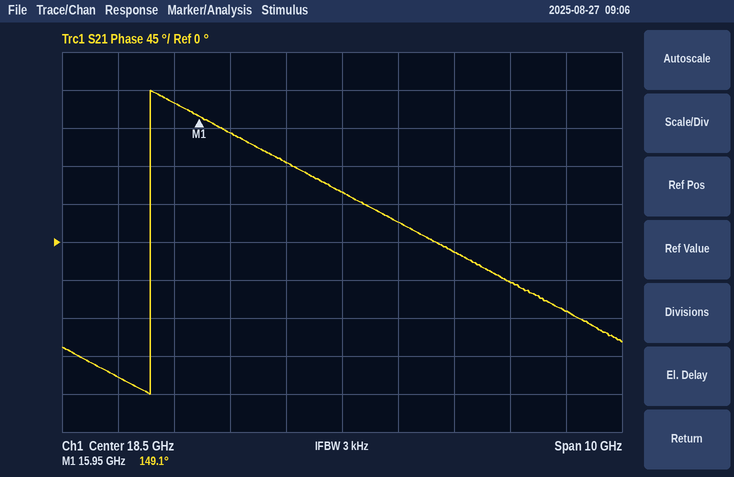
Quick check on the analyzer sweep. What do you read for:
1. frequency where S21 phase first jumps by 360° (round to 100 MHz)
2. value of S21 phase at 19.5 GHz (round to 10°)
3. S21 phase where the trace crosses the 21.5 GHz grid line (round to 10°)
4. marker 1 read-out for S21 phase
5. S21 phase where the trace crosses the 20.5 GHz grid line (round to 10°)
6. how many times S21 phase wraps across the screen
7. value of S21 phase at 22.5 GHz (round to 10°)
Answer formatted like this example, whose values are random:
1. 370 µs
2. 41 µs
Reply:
1. 15.1 GHz
2. 20°
3. -50°
4. 149.1°
5. -10°
6. 1
7. -80°
